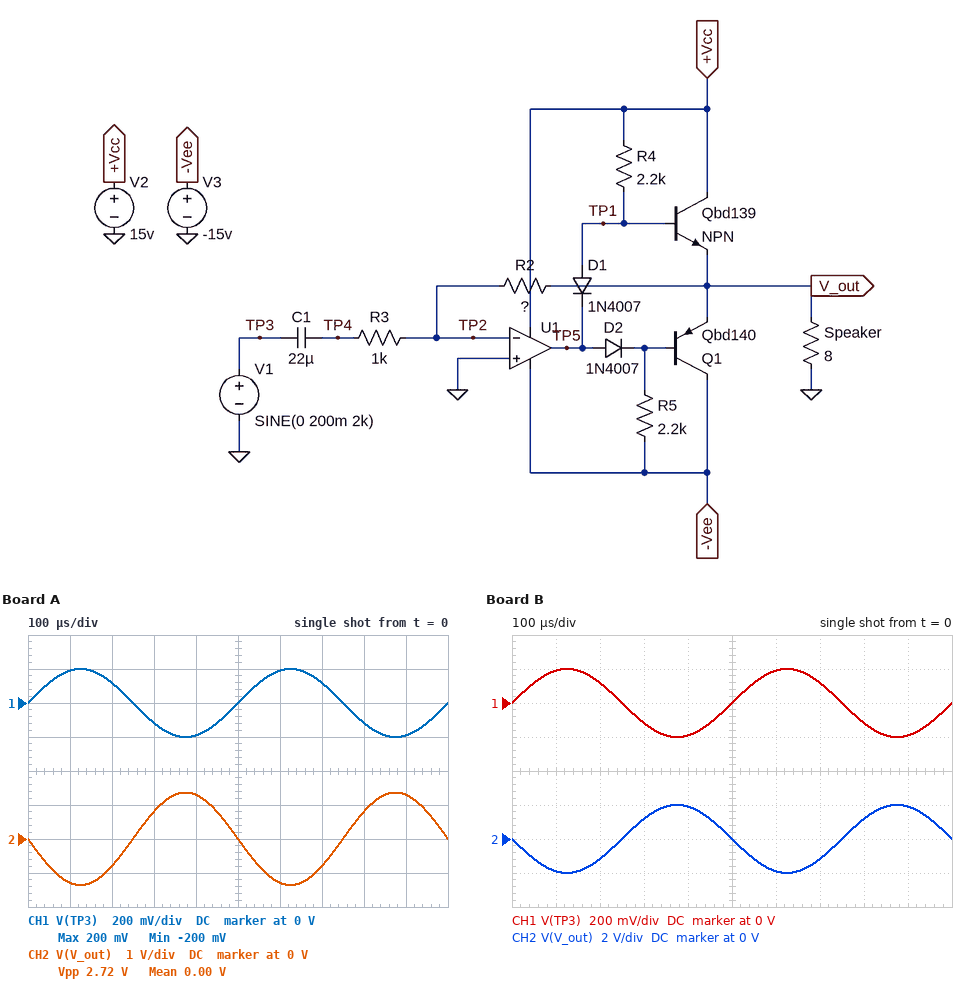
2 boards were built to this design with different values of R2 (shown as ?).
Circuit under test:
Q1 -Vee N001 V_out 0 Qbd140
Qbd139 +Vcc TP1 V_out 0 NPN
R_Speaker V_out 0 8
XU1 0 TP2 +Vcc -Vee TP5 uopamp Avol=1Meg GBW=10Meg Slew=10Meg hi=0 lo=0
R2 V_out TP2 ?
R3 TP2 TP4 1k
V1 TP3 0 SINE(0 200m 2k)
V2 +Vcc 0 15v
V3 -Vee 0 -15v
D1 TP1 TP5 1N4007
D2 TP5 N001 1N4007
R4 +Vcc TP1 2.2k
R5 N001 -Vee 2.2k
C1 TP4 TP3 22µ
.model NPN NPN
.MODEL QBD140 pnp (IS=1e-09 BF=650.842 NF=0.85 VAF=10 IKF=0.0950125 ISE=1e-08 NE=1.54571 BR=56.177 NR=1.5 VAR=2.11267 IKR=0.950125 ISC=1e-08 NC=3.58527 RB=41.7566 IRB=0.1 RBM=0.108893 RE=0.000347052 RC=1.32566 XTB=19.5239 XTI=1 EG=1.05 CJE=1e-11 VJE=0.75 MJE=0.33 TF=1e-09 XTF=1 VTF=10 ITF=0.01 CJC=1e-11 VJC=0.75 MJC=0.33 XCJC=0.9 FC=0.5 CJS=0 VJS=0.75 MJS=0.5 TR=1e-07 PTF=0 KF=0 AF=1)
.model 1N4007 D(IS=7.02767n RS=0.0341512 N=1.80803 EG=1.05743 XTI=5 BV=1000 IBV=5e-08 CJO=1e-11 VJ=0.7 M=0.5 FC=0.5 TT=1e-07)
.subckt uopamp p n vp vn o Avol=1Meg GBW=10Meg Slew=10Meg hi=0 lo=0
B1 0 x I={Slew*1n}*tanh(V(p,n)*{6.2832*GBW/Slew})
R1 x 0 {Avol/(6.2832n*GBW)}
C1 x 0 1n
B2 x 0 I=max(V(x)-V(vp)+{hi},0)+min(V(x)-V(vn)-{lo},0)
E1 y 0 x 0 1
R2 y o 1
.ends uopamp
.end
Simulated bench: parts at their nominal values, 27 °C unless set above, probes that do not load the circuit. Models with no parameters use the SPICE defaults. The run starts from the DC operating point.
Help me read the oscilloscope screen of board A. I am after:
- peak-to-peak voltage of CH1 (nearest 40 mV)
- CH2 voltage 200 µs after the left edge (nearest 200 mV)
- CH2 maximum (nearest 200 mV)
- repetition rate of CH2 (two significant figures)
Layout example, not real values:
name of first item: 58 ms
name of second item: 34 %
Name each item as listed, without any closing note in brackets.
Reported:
peak-to-peak voltage of CH1: 400 mV
CH2 voltage 200 µs after the left edge: -800 mV
CH2 maximum: 1.4 V
repetition rate of CH2: 2.0 kHz
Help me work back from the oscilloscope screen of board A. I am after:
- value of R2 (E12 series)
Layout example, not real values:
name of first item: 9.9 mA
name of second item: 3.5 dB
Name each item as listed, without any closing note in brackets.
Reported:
value of R2: 6.8 kΩ
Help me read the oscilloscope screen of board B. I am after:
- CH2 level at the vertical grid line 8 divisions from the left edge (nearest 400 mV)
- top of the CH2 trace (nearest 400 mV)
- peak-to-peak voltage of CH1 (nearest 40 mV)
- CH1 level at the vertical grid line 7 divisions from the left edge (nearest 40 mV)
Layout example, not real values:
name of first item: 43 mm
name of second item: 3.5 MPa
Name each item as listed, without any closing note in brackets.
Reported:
CH2 level at the vertical grid line 8 divisions from the left edge: 1.2 V
top of the CH2 trace: 2.0 V
peak-to-peak voltage of CH1: 400 mV
CH1 level at the vertical grid line 7 divisions from the left edge: 120 mV
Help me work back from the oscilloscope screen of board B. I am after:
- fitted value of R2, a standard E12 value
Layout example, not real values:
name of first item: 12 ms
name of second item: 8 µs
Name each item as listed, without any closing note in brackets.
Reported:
fitted value of R2, a standard E12 value: 10 kΩ
